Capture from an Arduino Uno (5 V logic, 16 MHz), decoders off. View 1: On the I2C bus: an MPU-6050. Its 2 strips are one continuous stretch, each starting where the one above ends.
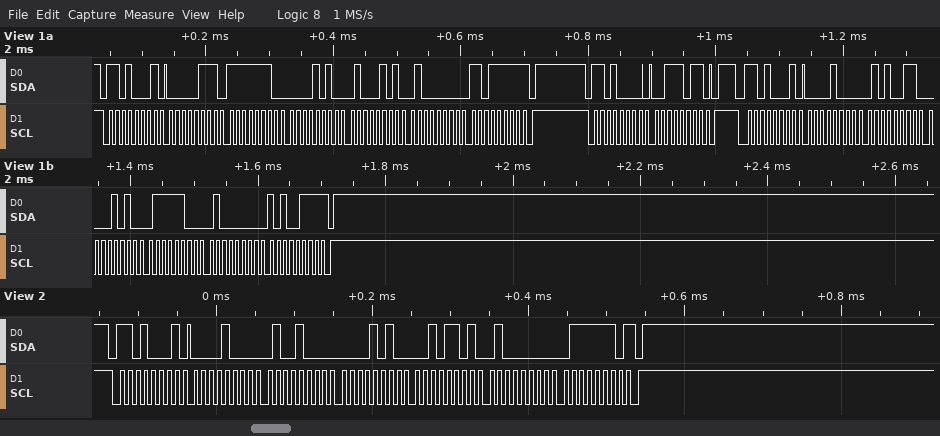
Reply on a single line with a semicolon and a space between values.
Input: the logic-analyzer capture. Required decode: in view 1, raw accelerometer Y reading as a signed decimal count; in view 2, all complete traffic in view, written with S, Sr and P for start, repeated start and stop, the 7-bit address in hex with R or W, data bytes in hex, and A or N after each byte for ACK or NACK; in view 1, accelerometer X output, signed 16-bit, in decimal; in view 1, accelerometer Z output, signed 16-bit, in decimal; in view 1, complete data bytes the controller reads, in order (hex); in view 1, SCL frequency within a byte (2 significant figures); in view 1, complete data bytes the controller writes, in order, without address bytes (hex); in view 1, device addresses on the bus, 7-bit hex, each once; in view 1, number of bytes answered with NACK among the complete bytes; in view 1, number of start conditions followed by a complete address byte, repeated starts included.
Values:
2684; S 68R A 08 A 48 A 0A A 2D A 40 A 7E N P; 2131; 16551; 07 FE 0A 45 40 DF 08 53 0A 7C 40 A7; 100 kHz; 3B; 0x68; 2; 3
